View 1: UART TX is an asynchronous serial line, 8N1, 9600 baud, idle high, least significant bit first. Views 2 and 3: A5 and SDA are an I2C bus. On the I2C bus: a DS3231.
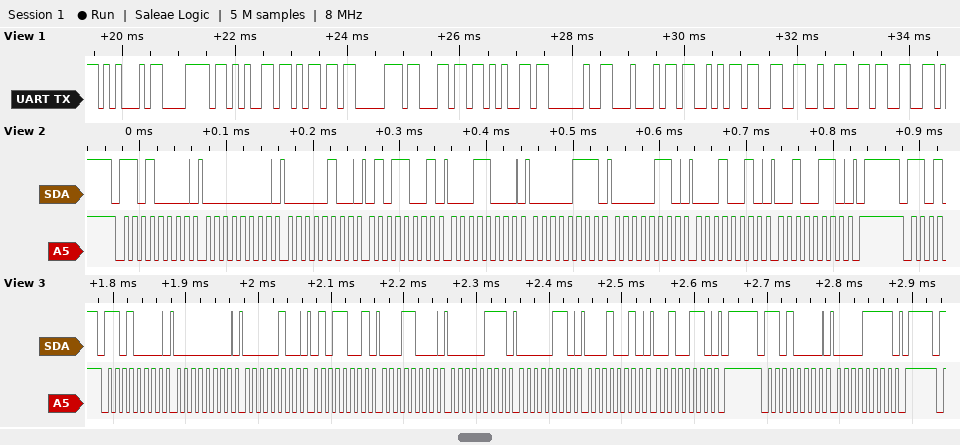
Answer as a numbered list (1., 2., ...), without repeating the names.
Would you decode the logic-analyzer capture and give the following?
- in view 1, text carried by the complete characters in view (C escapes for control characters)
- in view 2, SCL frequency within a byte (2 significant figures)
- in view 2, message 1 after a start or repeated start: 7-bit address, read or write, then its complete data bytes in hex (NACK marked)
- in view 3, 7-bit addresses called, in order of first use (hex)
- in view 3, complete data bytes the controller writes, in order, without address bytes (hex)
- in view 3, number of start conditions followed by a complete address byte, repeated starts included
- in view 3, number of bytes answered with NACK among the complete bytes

1. "Exemple DS323"
2. 100 kHz
3. 0x68 write: 00 04 59 18 07 06 12 26
4. 0x68
5. 00 04 59 18 07 06 12 26 0F
6. 2
7. 0
